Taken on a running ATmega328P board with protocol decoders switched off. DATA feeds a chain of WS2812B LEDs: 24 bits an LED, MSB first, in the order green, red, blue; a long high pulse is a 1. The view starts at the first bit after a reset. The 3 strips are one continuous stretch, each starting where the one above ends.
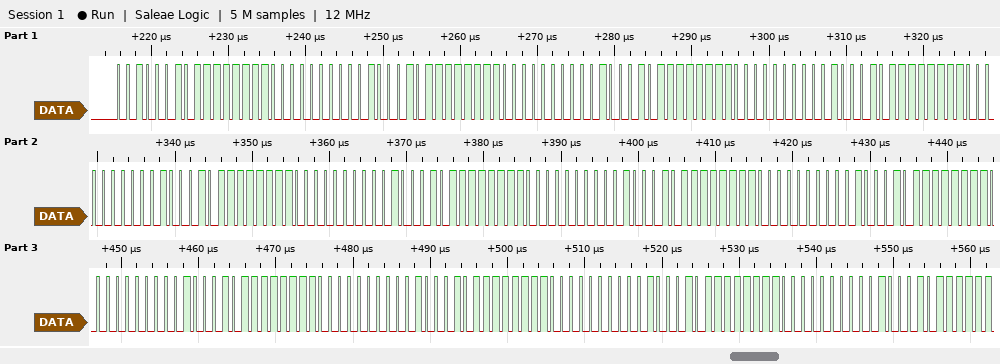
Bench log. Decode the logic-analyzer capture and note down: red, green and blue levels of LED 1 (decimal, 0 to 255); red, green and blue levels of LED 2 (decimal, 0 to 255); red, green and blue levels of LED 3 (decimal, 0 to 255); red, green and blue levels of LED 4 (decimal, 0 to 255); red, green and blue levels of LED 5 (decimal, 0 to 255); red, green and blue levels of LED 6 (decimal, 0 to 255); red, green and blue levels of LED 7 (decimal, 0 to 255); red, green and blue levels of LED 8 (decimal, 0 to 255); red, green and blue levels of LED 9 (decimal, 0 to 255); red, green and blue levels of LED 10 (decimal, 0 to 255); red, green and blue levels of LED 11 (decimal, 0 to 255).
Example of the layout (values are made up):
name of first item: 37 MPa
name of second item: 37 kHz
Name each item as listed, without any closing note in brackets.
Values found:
red, green and blue levels of LED 1: 255, 34, 0
red, green and blue levels of LED 2: 255, 34, 0
red, green and blue levels of LED 3: 255, 34, 0
red, green and blue levels of LED 4: 255, 34, 0
red, green and blue levels of LED 5: 255, 34, 0
red, green and blue levels of LED 6: 255, 34, 0
red, green and blue levels of LED 7: 255, 34, 0
red, green and blue levels of LED 8: 255, 34, 0
red, green and blue levels of LED 9: 255, 34, 0
red, green and blue levels of LED 10: 255, 34, 0
red, green and blue levels of LED 11: 255, 34, 0
